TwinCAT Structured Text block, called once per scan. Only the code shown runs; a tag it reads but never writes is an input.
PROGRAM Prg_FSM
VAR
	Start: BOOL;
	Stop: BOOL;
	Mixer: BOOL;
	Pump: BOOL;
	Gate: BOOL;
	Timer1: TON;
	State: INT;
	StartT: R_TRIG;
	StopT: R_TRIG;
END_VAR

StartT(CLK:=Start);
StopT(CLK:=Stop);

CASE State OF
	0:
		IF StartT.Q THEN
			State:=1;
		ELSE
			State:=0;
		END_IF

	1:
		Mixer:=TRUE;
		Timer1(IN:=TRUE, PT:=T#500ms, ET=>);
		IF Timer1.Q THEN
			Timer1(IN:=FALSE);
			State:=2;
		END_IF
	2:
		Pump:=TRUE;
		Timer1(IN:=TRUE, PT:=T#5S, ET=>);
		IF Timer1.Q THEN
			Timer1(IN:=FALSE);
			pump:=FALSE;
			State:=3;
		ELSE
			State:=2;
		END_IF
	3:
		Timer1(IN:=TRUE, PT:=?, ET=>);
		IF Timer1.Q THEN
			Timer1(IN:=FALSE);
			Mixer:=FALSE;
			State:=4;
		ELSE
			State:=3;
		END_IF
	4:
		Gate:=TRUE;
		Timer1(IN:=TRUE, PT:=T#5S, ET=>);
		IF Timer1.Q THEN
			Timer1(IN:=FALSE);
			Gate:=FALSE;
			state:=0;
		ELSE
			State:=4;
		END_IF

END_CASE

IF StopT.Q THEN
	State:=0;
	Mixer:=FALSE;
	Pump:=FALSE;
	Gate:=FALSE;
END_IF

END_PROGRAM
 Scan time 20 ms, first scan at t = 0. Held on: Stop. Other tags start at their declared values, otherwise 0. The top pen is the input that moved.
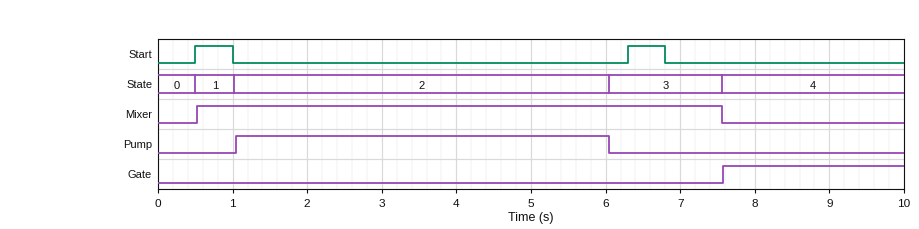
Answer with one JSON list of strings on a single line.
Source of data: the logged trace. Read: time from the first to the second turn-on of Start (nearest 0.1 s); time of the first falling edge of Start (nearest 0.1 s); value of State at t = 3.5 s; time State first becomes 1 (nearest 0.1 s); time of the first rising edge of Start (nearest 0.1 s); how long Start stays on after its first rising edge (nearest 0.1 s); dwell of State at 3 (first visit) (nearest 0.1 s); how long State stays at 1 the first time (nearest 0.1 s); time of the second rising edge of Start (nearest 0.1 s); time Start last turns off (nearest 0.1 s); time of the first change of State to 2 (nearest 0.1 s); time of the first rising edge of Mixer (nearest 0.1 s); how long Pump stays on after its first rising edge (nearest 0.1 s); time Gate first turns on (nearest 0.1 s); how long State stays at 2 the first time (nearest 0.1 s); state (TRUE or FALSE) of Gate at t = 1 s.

["5.8 s", "1.0 s", "2", "0.5 s", "0.5 s", "0.5 s", "1.5 s", "0.5 s", "6.3 s", "6.8 s", "1.0 s", "0.5 s", "5.0 s", "7.6 s", "5.0 s", "FALSE"]
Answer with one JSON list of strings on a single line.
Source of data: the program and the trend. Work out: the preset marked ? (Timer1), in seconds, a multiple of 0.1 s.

["1.5 s"]
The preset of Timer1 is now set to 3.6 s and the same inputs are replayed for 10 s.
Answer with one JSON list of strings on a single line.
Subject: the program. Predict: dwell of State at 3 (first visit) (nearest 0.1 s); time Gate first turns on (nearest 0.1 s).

["3.6 s", "9.7 s"]
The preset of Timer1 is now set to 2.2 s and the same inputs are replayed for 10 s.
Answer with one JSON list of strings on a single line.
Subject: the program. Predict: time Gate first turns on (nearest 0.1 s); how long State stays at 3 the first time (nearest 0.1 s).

["8.3 s", "2.2 s"]
